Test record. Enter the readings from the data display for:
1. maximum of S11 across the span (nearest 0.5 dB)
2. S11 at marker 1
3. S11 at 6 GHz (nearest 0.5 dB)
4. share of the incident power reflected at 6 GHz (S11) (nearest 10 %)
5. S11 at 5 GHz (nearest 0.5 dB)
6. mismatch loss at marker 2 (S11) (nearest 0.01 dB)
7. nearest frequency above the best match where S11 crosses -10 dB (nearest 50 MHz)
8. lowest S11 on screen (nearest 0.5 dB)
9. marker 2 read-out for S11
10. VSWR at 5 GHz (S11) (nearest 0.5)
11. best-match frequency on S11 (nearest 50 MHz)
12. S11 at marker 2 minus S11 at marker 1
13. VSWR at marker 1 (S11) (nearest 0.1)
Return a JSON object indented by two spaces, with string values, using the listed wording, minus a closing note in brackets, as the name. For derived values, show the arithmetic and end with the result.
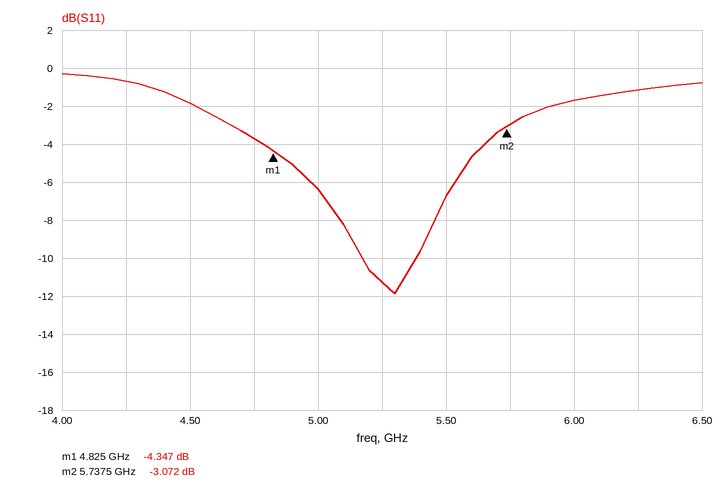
{
  "maximum of S11 across the span": "-0.5 dB",
  "S11 at marker 1": "-4.347 dB",
  "S11 at 6 GHz": "-1.5 dB",
  "share of the incident power reflected at 6 GHz (S11)": "10^(-1.5/10) ≈ 70.8 %, so 70 % to the nearest 10 %",
  "S11 at 5 GHz": "-6.5 dB",
  "mismatch loss at marker 2 (S11)": "−10 log10(1 − 10^(-3.072/10)) ≈ 2.95 dB",
  "nearest frequency above the best match where S11 crosses -10 dB": "5.40 GHz",
  "lowest S11 on screen": "-12.0 dB",
  "marker 2 read-out for S11": "-3.072 dB",
  "VSWR at 5 GHz (S11)": "|Γ| = 10^(-6.5/20) = 0.4732; VSWR = (1 + 0.4732)/(1 − 0.4732) ≈ 2.80, so 3.0 to the nearest 0.5",
  "best-match frequency on S11": "5.30 GHz",
  "S11 at marker 2 minus S11 at marker 1": "-3.072 − (-4.347) = 1.275 dB",
  "VSWR at marker 1 (S11)": "(1 + 0.6062)/(1 − 0.6062) ≈ 4.1"
}
